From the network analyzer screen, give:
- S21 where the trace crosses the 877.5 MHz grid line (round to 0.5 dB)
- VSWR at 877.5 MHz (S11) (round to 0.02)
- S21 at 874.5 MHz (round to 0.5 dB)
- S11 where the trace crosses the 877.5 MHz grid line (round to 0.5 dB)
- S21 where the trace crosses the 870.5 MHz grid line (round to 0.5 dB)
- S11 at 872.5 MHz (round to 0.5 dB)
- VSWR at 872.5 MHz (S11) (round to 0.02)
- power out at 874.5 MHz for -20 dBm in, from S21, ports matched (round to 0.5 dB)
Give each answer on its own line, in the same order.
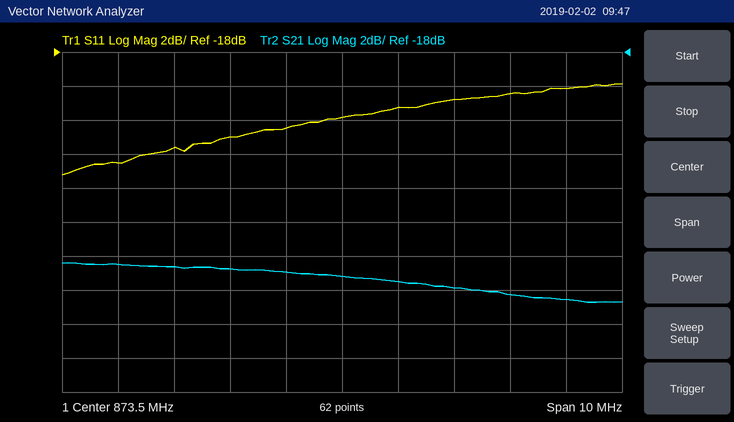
-32.5 dB
1.22
-31.5 dB
-20.0 dB
-30.5 dB
-22.5 dB
1.16
-51.5 dBm
